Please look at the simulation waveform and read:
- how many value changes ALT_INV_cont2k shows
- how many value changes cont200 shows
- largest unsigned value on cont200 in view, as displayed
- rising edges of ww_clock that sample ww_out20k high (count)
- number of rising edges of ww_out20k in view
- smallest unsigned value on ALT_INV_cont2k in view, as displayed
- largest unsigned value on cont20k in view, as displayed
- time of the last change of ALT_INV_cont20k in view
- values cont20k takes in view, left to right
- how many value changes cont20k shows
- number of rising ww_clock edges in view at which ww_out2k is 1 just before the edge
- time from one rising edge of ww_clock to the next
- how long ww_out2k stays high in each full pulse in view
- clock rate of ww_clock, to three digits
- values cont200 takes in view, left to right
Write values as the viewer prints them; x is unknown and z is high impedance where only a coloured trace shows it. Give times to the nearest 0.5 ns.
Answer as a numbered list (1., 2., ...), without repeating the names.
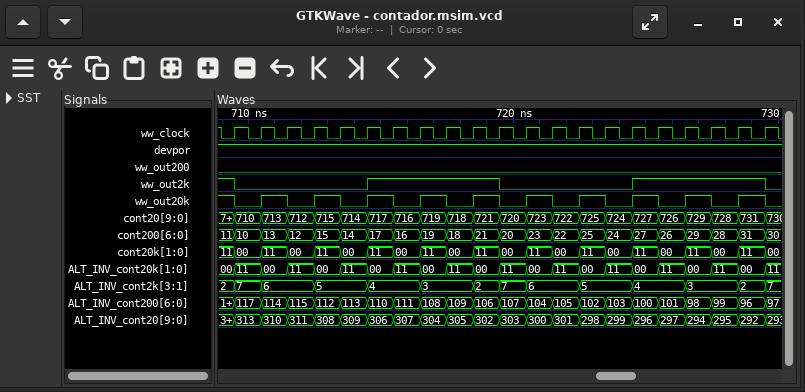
1. 13
2. 21
3. 31
4. 11
5. 10
6. 2
7. 11
8. 729.5 ns
9. 11, 00, 11, 00, 11, 00, 11, 00, 11, 00, 11, 00, 11, 00, 11, 00, 11, 00, 11, 00, 11, 00
10. 21
11. 11
12. 1 ns
13. 5 ns, 5 ns
14. 1.00 GHz
15. 11, 10, 13, 12, 15, 14, 17, 16, 19, 18, 21, 20, 23, 22, 25, 24, 27, 26, 29, 28, 31, 30
